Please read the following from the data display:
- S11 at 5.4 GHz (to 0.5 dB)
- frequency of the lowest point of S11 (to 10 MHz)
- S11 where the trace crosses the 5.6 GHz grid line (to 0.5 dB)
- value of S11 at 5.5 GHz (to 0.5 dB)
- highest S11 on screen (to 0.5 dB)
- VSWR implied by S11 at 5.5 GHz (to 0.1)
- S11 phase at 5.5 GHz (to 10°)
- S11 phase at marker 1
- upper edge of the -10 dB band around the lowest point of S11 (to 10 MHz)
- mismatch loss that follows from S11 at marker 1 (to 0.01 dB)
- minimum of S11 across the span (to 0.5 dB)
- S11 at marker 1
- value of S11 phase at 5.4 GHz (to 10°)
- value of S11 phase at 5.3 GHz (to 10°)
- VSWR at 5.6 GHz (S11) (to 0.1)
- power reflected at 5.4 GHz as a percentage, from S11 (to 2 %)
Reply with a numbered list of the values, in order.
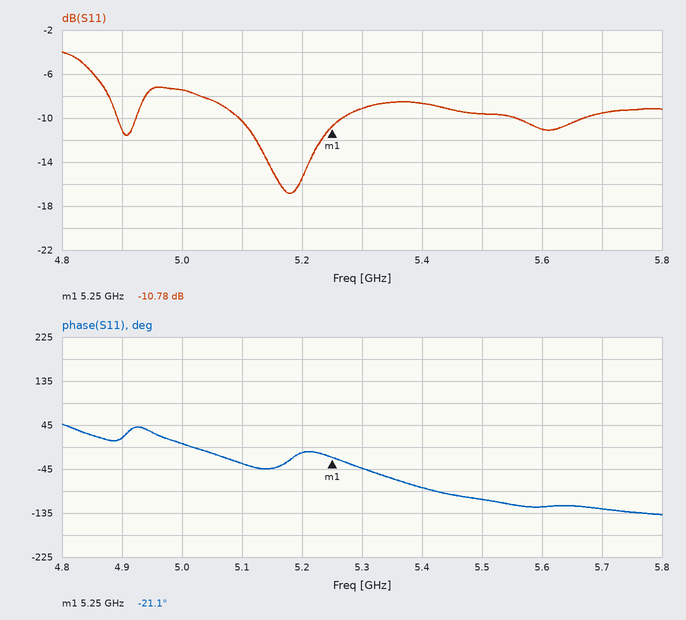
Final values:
1. -8.5 dB
2. 5.18 GHz
3. -11.0 dB
4. -9.5 dB
5. -4.0 dB
6. 2.0
7. -110°
8. -21.1°
9. 5.27 GHz
10. 0.38 dB
11. -17.0 dB
12. -10.78 dB
13. -80°
14. -40°
15. 1.8
16. 14 %
